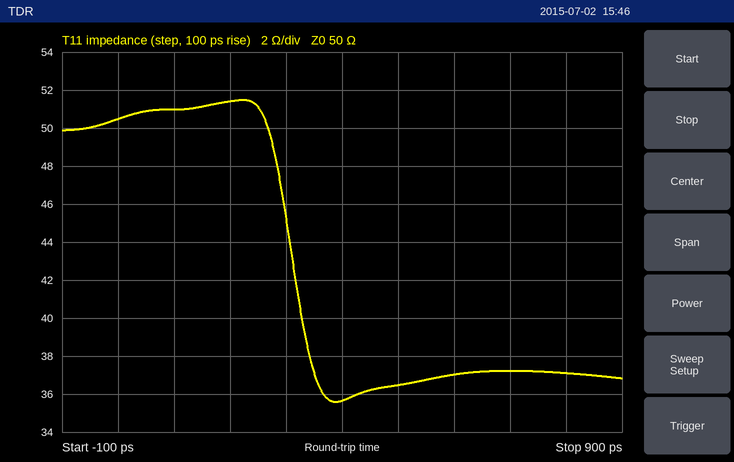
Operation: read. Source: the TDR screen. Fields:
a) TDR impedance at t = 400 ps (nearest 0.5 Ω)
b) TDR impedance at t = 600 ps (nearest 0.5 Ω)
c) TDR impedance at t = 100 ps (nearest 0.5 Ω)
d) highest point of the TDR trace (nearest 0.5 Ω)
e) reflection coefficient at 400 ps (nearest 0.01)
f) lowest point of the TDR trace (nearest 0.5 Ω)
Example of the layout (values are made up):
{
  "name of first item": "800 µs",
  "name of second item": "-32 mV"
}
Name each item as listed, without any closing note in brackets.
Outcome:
{
  "TDR impedance at t = 400 ps": "35.5 Ω",
  "TDR impedance at t = 600 ps": "37.0 Ω",
  "TDR impedance at t = 100 ps": "51.0 Ω",
  "highest point of the TDR trace": "51.5 Ω",
  "reflection coefficient at 400 ps": "-0.17",
  "lowest point of the TDR trace": "35.5 Ω"
}
